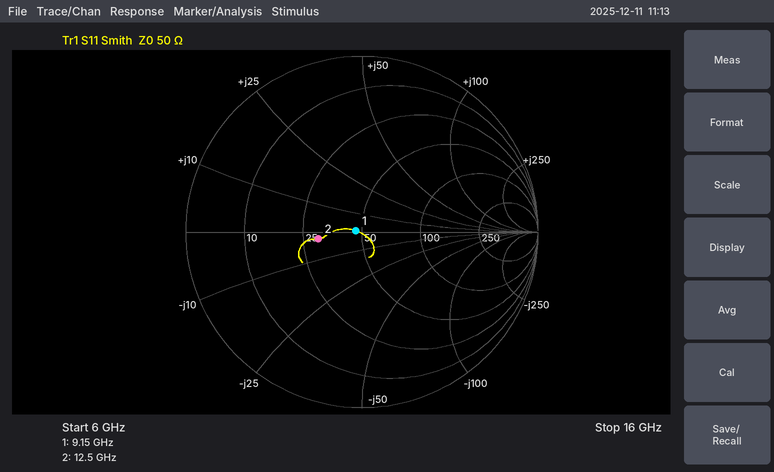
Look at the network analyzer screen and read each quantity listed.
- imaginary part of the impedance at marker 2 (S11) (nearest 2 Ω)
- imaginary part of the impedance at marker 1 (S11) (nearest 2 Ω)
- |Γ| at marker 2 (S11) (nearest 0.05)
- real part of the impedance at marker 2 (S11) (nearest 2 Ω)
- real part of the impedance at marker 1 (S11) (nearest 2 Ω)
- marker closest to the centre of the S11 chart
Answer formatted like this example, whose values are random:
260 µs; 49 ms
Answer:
-2 Ω; 0 Ω; 0.25; 30 Ω; 46 Ω; marker 1
